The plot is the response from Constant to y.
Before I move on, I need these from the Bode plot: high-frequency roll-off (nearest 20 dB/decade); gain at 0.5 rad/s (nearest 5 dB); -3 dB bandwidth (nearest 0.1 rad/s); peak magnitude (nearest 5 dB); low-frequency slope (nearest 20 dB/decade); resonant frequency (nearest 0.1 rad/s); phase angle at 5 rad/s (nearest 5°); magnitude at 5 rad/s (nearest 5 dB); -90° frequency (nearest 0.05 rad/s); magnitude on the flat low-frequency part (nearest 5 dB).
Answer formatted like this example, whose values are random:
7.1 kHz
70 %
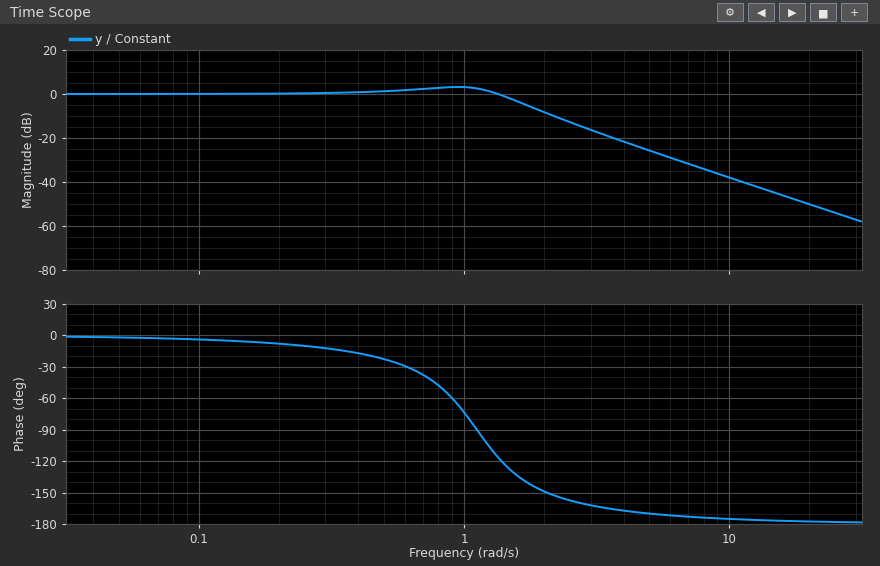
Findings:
-40 dB/decade
0 dB
1.6 rad/s
5 dB
0 dB/decade
0.9 rad/s
-170°
-25 dB
1.10 rad/s
0 dB
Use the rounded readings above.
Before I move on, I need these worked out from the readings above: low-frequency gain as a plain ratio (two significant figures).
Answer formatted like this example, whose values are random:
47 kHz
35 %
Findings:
1.0
